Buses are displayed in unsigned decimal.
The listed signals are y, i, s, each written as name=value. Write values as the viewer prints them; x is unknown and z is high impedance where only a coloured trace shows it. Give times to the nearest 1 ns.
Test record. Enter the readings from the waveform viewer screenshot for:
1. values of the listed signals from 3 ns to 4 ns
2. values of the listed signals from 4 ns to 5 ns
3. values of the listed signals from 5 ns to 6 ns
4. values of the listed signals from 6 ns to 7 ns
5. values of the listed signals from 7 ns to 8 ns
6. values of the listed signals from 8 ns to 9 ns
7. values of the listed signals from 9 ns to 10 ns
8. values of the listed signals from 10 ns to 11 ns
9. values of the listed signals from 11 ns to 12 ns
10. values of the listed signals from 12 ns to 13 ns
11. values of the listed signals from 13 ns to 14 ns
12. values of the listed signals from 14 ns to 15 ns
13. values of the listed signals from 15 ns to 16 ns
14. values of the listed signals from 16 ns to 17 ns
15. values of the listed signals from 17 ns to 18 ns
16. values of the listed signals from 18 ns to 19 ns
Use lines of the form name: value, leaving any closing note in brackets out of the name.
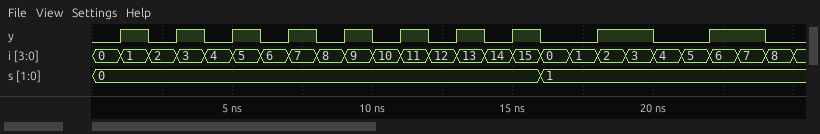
values of the listed signals from 3 ns to 4 ns: y=1, i=3, s=0
values of the listed signals from 4 ns to 5 ns: y=0, i=4, s=0
values of the listed signals from 5 ns to 6 ns: y=1, i=5, s=0
values of the listed signals from 6 ns to 7 ns: y=0, i=6, s=0
values of the listed signals from 7 ns to 8 ns: y=1, i=7, s=0
values of the listed signals from 8 ns to 9 ns: y=0, i=8, s=0
values of the listed signals from 9 ns to 10 ns: y=1, i=9, s=0
values of the listed signals from 10 ns to 11 ns: y=0, i=10, s=0
values of the listed signals from 11 ns to 12 ns: y=1, i=11, s=0
values of the listed signals from 12 ns to 13 ns: y=0, i=12, s=0
values of the listed signals from 13 ns to 14 ns: y=1, i=13, s=0
values of the listed signals from 14 ns to 15 ns: y=0, i=14, s=0
values of the listed signals from 15 ns to 16 ns: y=1, i=15, s=0
values of the listed signals from 16 ns to 17 ns: y=0, i=0, s=1
values of the listed signals from 17 ns to 18 ns: y=0, i=1, s=1
values of the listed signals from 18 ns to 19 ns: y=1, i=2, s=1
